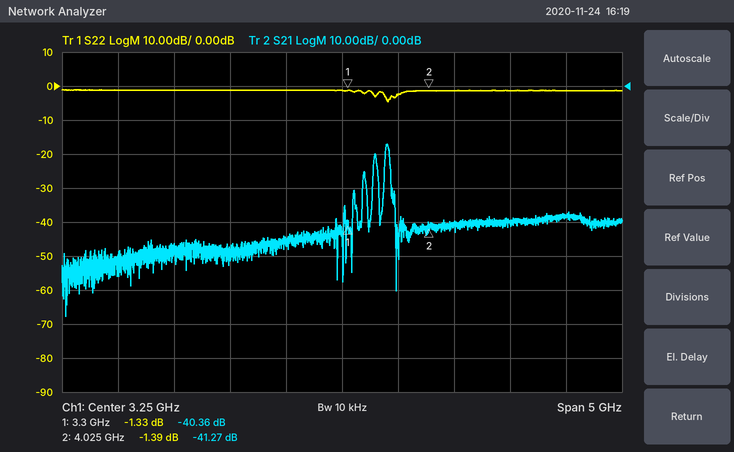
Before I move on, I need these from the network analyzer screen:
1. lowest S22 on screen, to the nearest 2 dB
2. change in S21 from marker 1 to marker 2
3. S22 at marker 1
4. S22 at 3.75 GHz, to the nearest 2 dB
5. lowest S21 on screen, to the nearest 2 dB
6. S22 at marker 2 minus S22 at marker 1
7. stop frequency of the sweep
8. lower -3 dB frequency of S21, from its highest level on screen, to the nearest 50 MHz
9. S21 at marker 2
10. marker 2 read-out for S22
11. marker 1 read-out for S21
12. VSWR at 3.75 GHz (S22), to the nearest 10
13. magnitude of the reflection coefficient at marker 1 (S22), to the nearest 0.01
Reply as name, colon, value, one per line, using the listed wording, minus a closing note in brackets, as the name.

lowest S22 on screen, to the nearest 2 dB: -4 dB
change in S21 from marker 1 to marker 2: -0.91 dB
S22 at marker 1: -1.33 dB
S22 at 3.75 GHz, to the nearest 2 dB: -2 dB
lowest S21 on screen, to the nearest 2 dB: -68 dB
S22 at marker 2 minus S22 at marker 1: -0.06 dB
stop frequency of the sweep: 5.75 GHz
lower -3 dB frequency of S21, from its highest level on screen, to the nearest 50 MHz: 3.65 GHz
S21 at marker 2: -41.27 dB
marker 2 read-out for S22: -1.39 dB
marker 1 read-out for S21: -40.36 dB
VSWR at 3.75 GHz (S22), to the nearest 10: 10
magnitude of the reflection coefficient at marker 1 (S22), to the nearest 0.01: 0.86
